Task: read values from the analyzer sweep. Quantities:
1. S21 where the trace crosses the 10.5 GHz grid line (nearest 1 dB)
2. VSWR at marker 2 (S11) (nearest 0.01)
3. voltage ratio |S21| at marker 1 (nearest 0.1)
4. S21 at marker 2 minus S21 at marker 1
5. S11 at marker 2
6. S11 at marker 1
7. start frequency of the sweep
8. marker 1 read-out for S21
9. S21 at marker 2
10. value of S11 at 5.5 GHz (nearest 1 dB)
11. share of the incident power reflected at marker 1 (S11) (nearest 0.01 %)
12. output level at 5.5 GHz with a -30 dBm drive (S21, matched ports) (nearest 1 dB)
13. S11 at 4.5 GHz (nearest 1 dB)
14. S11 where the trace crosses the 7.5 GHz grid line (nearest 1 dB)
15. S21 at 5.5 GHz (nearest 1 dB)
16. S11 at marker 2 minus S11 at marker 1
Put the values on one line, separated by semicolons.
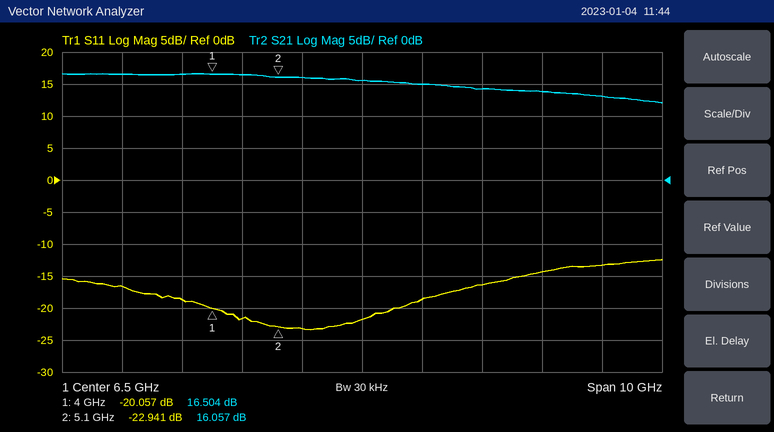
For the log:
13 dB; 1.15; 6.7; -0.447 dB; -22.941 dB; -20.057 dB; 1.5 GHz; 16.504 dB; 16.057 dB; -23 dB; 0.99 %; -14 dBm; -22 dB; -19 dB; 16 dB; -2.884 dB
